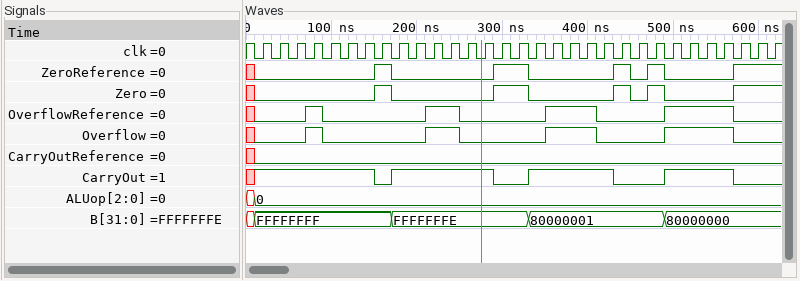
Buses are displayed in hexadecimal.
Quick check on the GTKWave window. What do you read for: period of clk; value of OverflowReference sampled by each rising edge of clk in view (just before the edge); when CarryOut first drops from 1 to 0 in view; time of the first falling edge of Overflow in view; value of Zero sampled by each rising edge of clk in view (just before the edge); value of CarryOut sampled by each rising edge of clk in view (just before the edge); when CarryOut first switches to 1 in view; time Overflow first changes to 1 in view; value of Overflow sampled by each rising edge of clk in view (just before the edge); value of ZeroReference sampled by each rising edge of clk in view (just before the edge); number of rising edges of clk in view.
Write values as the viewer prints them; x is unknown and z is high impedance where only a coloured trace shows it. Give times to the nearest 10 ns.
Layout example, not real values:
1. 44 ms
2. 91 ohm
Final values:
1. 20 ns
2. 0 0 0 1 0 0 0 0 0 0 1 1 0 0 0 0 0 1 1 1 0 0 0 0 1 1 1 1 0 0 0
3. 150 ns
4. 90 ns
5. 0 0 0 0 0 0 0 1 0 0 0 0 0 0 1 1 0 0 0 0 0 1 0 1 0 0 0 0 1 1 1
6. 1 1 1 1 1 1 1 0 1 1 1 1 1 1 0 0 1 1 1 1 1 0 0 0 1 1 1 1 0 0 0
7. 10 ns
8. 70 ns
9. 0 0 0 1 0 0 0 0 0 0 1 1 0 0 0 0 0 1 1 1 0 0 0 0 1 1 1 1 0 0 0
10. 0 0 0 0 0 0 0 1 0 0 0 0 0 0 1 1 0 0 0 0 0 1 0 1 0 0 0 0 1 1 1
11. 31
